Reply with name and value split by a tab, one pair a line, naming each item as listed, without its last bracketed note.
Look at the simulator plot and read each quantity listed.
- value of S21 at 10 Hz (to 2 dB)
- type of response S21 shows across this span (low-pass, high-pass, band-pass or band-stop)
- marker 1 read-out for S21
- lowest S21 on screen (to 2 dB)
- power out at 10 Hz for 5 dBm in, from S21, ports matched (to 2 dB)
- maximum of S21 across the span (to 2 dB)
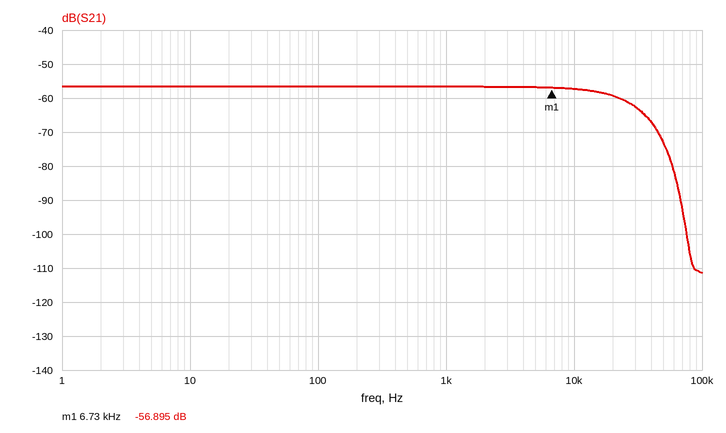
value of S21 at 10 Hz	-56 dB
type of response S21 shows across this span	low-pass
marker 1 read-out for S21	-56.895 dB
lowest S21 on screen	-112 dB
power out at 10 Hz for 5 dBm in, from S21, ports matched	-52 dBm
maximum of S21 across the span	-56 dB
